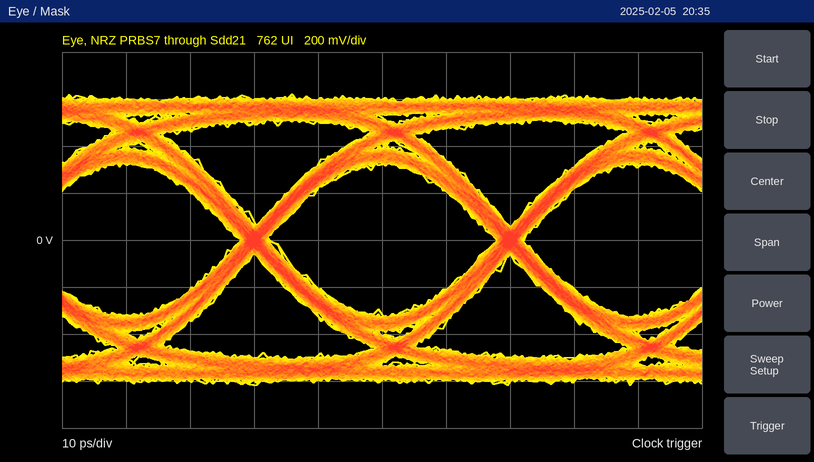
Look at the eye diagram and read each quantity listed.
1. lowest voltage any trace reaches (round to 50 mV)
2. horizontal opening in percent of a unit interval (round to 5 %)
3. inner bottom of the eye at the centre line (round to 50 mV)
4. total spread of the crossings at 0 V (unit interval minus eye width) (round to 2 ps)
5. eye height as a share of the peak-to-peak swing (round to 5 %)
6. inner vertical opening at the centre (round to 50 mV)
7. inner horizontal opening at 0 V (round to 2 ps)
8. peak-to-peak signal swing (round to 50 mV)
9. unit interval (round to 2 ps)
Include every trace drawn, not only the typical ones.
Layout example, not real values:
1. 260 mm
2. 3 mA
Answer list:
1. -600 mV
2. 90 %
3. -300 mV
4. 4 ps
5. 50 %
6. 650 mV
7. 36 ps
8. 1.25 V
9. 40 ps
